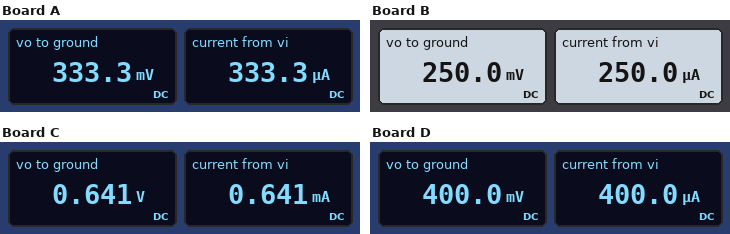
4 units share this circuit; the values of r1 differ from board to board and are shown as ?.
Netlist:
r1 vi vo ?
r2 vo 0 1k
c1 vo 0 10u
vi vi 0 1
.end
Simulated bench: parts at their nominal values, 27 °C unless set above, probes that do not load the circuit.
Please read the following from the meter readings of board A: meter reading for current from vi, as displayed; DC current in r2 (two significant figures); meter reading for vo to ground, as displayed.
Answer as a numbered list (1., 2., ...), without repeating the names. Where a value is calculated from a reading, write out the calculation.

1. 333.3 µA
2. (333.3 mV) / 1 kΩ = 330 µA
3. 333.3 mV
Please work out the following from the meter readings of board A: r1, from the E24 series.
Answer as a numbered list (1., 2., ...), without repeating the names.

1. 2 kΩ
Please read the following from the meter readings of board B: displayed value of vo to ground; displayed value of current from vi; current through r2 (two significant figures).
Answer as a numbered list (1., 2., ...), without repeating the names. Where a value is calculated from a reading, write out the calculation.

1. 250.0 mV
2. 250.0 µA
3. (250 mV) / 1 kΩ = 250 µA
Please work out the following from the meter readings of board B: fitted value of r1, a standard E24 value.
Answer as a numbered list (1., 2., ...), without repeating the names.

1. 3 kΩ
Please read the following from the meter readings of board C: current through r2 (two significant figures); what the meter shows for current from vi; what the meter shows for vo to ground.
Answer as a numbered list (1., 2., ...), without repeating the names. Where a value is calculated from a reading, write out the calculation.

1. (641 mV) / 1 kΩ = 640 µA
2. 0.641 mA
3. 0.641 V
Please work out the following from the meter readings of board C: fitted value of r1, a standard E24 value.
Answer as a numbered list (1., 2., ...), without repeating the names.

1. 560 Ω
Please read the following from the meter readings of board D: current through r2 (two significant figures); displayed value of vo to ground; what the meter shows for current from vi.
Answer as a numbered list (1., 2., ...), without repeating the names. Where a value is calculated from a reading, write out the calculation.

1. (400 mV) / 1 kΩ = 400 µA
2. 400.0 mV
3. 400.0 µA
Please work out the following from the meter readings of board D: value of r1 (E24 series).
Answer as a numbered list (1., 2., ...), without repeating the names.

1. 1.5 kΩ
